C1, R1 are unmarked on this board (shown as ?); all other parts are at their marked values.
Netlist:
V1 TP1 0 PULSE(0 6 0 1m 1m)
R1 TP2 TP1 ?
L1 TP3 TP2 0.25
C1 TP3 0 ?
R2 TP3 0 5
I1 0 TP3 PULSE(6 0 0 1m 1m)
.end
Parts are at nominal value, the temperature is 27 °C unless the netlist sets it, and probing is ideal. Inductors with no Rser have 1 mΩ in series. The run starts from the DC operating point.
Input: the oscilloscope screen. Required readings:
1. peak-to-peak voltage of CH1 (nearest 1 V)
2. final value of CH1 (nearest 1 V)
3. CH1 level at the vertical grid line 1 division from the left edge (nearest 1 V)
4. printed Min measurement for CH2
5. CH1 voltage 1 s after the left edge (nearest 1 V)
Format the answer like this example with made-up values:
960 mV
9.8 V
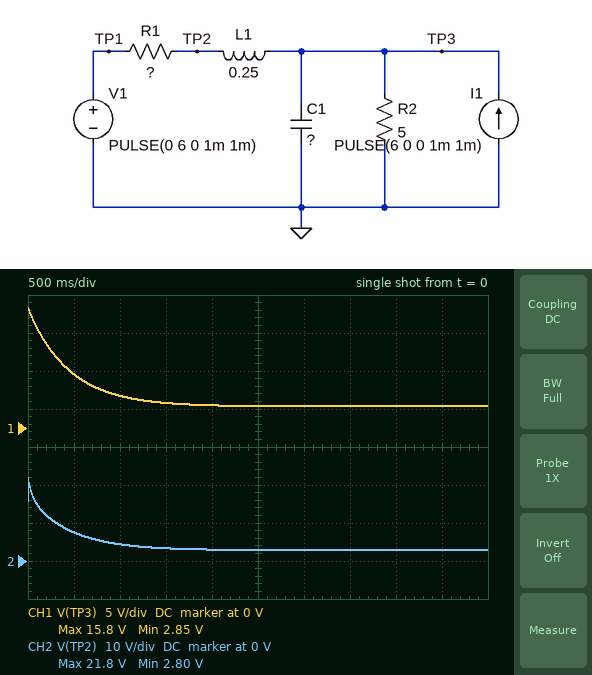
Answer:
13 V
3 V
7 V
2.80 V
4 V
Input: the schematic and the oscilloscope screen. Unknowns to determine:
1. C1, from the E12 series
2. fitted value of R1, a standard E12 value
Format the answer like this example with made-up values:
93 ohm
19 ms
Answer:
180 mF
5.6 Ω
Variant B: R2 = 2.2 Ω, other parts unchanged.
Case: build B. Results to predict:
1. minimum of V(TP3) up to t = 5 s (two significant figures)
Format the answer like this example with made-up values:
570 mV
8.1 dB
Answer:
1.7 V
